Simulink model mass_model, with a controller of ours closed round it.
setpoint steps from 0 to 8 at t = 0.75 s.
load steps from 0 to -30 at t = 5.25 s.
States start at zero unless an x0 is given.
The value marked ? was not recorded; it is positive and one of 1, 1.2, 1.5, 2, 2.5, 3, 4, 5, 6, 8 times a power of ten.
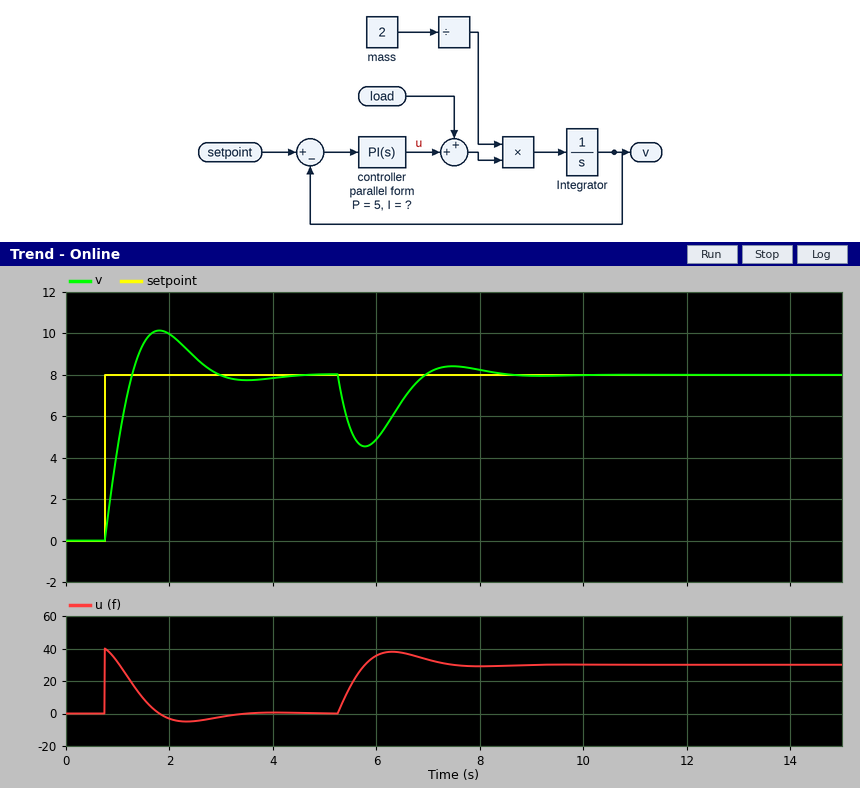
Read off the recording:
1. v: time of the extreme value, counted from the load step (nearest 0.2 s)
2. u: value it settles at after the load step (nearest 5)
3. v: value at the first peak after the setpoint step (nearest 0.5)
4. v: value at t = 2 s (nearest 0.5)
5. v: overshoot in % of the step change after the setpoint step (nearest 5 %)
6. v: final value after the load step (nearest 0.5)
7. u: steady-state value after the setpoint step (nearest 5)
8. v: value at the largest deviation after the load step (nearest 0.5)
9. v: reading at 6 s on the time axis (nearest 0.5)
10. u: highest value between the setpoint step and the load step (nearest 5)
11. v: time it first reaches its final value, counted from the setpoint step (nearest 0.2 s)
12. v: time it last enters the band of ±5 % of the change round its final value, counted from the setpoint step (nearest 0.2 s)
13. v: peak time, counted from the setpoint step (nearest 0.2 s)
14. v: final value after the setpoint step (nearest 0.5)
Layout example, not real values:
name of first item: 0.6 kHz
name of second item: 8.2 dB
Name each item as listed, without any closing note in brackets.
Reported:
v: time of the extreme value, counted from the load step: 0.6 s
u: value it settles at after the load step: 30
v: value at the first peak after the setpoint step: 10.0
v: value at t = 2 s: 10.0
v: overshoot in % of the step change after the setpoint step: 25 %
v: final value after the load step: 8.0
u: steady-state value after the setpoint step: 0
v: value at the largest deviation after the load step: 4.5
v: reading at 6 s on the time axis: 5.0
u: highest value between the setpoint step and the load step: 40
v: time it first reaches its final value, counted from the setpoint step: 0.6 s
v: time it last enters the band of ±5 % of the change round its final value, counted from the setpoint step: 2.0 s
v: peak time, counted from the setpoint step: 1.0 s
v: final value after the setpoint step: 8.0
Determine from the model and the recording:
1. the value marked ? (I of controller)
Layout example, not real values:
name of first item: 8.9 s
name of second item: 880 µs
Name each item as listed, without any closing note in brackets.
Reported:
the value marked ?: 10
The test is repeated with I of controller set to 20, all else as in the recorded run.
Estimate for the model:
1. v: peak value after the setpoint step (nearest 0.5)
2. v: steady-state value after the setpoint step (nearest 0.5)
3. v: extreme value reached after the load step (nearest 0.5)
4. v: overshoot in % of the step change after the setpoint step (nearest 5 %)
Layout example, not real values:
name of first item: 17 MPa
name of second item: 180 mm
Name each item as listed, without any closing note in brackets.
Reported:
v: peak value after the setpoint step: 11.0
v: steady-state value after the setpoint step: 8.0
v: extreme value reached after the load step: 5.0
v: overshoot in % of the step change after the setpoint step: 35 %
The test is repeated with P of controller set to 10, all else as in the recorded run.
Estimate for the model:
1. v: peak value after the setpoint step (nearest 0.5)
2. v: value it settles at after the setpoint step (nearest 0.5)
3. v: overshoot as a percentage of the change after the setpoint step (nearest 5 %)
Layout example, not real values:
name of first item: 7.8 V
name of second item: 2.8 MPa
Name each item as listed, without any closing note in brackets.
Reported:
v: peak value after the setpoint step: 9.0
v: value it settles at after the setpoint step: 8.0
v: overshoot as a percentage of the change after the setpoint step: 10 %
